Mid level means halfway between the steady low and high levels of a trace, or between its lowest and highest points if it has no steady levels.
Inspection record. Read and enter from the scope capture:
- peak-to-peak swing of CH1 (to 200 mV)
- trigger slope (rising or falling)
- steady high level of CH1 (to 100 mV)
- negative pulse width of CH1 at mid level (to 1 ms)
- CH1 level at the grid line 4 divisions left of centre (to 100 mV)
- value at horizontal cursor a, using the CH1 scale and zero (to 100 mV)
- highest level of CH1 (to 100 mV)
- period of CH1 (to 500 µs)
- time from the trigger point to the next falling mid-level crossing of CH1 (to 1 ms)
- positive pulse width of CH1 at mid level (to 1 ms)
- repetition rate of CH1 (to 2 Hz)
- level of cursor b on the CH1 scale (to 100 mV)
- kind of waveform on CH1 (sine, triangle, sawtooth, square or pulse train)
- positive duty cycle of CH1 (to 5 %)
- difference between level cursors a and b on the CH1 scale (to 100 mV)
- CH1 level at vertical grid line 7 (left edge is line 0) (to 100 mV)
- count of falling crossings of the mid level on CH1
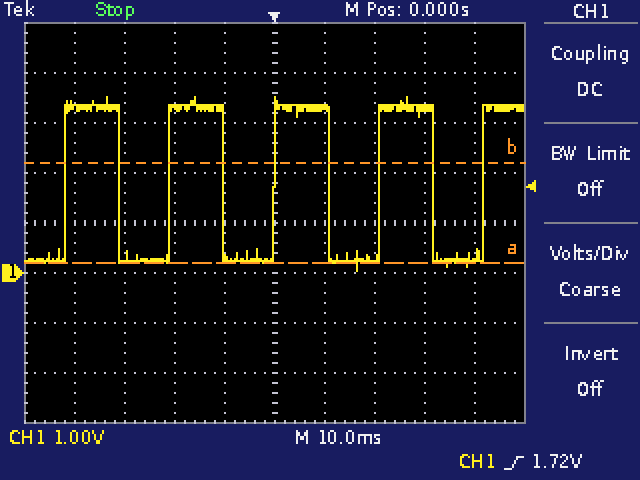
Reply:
3.4 V
rising
3.3 V
10 ms
3.3 V
200 mV
3.5 V
21.0 ms
11 ms
11 ms
48 Hz
2.2 V
square
50 %
2.0 V
300 mV
4
